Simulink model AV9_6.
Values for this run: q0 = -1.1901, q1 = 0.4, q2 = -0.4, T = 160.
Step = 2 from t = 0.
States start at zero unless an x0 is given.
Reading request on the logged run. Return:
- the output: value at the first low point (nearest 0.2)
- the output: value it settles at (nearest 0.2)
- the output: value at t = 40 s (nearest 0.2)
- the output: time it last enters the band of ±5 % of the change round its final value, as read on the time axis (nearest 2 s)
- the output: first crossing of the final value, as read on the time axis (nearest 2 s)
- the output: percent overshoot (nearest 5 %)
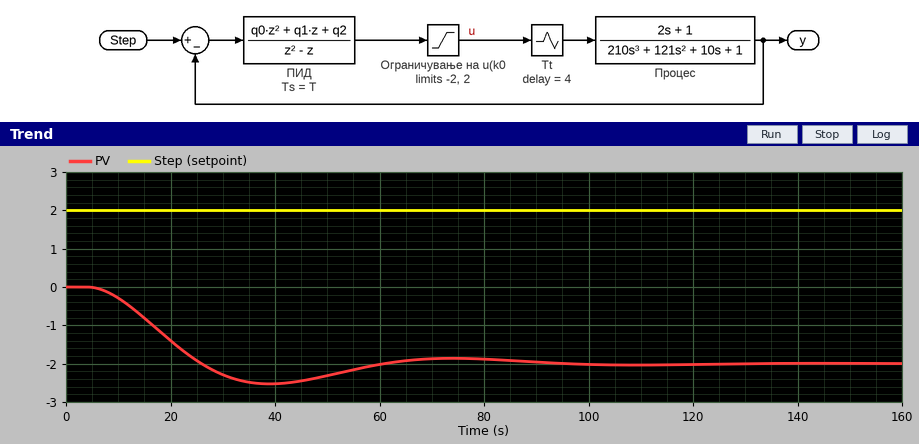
-2.6
-2.0
-2.6
82 s
26 s
25 %
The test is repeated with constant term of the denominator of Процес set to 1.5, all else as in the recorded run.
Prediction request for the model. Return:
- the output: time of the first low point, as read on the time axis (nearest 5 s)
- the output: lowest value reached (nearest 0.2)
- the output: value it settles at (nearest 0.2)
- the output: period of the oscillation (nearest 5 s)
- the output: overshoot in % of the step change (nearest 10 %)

30 s
-1.8
-1.4
55 s
40 %
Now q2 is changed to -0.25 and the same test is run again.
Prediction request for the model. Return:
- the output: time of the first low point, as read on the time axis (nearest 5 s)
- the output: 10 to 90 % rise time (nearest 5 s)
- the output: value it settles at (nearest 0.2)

40 s
15 s
-2.0
